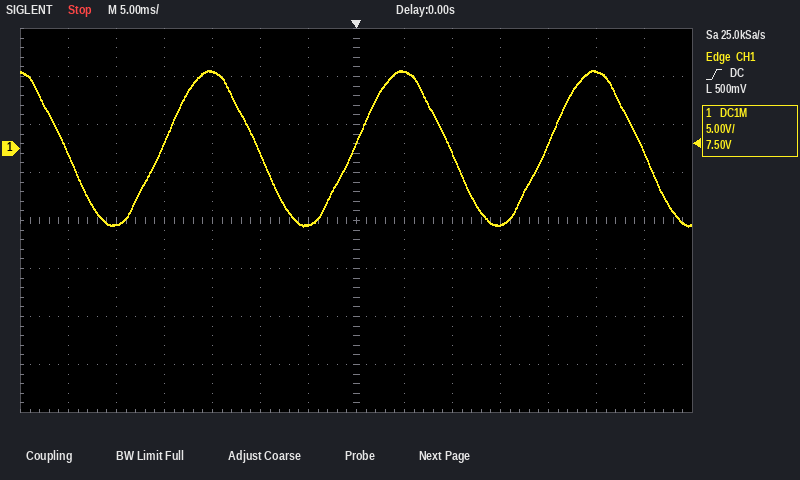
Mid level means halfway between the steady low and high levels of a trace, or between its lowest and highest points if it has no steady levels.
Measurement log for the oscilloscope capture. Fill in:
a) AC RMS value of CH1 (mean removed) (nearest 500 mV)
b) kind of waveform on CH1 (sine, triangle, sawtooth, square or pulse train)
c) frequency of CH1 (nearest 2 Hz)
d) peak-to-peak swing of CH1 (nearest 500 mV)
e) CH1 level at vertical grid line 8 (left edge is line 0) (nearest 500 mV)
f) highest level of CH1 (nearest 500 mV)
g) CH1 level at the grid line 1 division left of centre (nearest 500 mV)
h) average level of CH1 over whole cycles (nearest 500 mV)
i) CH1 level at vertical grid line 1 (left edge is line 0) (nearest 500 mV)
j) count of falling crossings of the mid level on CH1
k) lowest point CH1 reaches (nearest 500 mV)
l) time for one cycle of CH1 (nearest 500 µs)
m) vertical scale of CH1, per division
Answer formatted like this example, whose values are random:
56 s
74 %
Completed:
5.5 V
sine
50 Hz
16.0 V
8.0 V
8.0 V
-8.0 V
0.0 V
-500 mV
4
-8.0 V
20.0 ms
5 V
